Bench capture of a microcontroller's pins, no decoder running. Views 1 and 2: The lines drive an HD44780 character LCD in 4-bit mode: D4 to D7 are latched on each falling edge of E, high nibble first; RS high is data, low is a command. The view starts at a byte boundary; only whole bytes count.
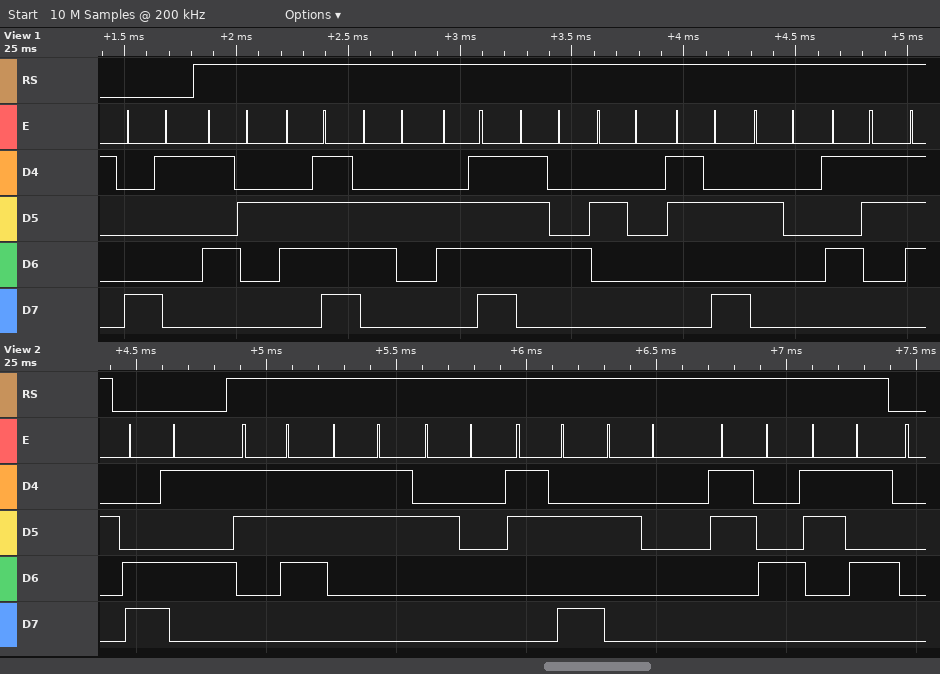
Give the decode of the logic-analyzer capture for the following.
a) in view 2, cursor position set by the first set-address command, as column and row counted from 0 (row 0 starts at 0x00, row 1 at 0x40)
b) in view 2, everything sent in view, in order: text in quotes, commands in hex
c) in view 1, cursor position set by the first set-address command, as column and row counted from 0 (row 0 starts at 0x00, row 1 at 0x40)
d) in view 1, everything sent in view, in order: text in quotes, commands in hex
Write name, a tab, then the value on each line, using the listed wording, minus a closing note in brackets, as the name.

in view 2, cursor position set by the first set-address command, as column and row counted from 0	column 5, row 1
in view 2, everything sent in view, in order: text in quotes, commands in hex	0xC5 "73 : 45"
in view 1, cursor position set by the first set-address command, as column and row counted from 0	column 1, row 0
in view 1, everything sent in view, in order: text in quotes, commands in hex	0x81 "Robot : S"
